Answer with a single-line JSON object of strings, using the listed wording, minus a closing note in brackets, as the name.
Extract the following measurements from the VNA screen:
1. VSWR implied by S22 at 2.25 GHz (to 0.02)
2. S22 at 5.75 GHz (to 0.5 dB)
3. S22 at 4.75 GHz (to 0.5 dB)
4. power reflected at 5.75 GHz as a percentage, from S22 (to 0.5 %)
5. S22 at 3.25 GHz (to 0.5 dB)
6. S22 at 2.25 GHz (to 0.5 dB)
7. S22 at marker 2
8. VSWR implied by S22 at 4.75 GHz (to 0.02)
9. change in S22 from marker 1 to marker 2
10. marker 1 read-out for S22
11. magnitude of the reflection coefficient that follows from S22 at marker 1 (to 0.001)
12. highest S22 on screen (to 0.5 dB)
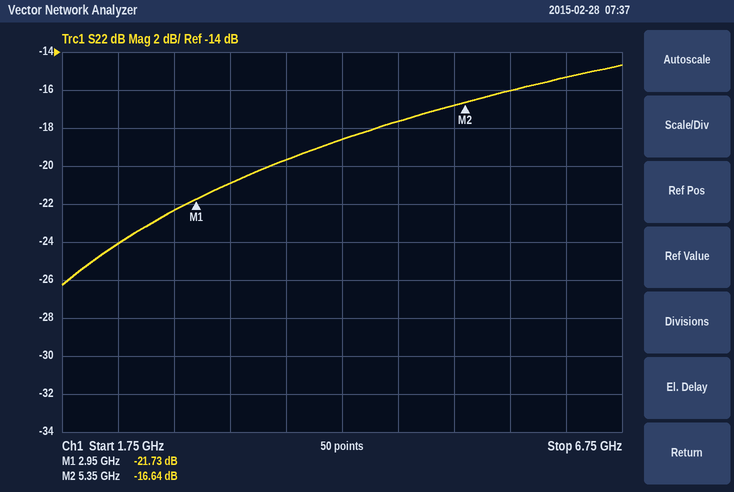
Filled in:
{"VSWR implied by S22 at 2.25 GHz": "1.14", "S22 at 5.75 GHz": "-16.0 dB", "S22 at 4.75 GHz": "-17.5 dB", "power reflected at 5.75 GHz as a percentage, from S22": "2.5 %", "S22 at 3.25 GHz": "-21.0 dB", "S22 at 2.25 GHz": "-24.0 dB", "S22 at marker 2": "-16.64 dB", "VSWR implied by S22 at 4.75 GHz": "1.30", "change in S22 from marker 1 to marker 2": "5.09 dB", "marker 1 read-out for S22": "-21.73 dB", "magnitude of the reflection coefficient that follows from S22 at marker 1": "0.082", "highest S22 on screen": "-14.5 dB"}
